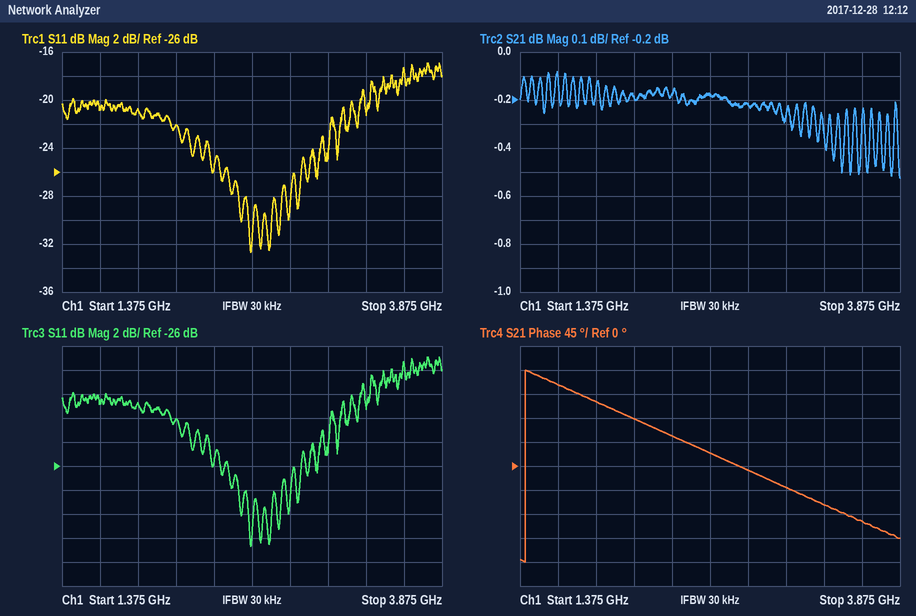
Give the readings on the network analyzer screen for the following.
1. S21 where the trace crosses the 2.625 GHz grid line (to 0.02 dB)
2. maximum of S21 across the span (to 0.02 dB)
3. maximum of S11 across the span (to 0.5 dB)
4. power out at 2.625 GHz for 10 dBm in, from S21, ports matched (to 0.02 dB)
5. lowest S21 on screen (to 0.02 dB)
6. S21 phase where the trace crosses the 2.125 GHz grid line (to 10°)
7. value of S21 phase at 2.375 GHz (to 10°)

-0.18 dB
-0.08 dB
-17.0 dB
9.82 dBm
-0.52 dB
90°
60°
